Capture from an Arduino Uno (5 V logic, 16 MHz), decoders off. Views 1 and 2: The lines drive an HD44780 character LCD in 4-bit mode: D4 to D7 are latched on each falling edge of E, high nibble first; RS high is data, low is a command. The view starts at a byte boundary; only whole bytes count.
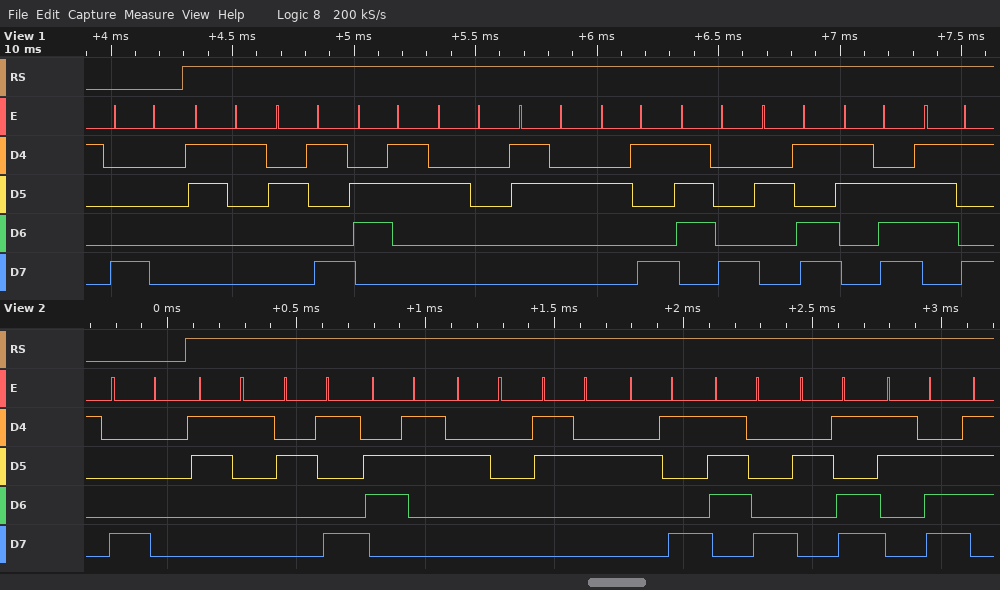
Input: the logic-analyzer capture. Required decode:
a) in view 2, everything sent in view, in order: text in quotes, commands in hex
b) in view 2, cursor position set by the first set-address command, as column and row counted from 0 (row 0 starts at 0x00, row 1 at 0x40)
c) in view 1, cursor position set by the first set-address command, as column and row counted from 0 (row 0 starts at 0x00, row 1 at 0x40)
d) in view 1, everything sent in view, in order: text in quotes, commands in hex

0x80 "1)c 2)x->"
column 0, row 0
column 0, row 0
0x80 "1)c 2)x->y"
